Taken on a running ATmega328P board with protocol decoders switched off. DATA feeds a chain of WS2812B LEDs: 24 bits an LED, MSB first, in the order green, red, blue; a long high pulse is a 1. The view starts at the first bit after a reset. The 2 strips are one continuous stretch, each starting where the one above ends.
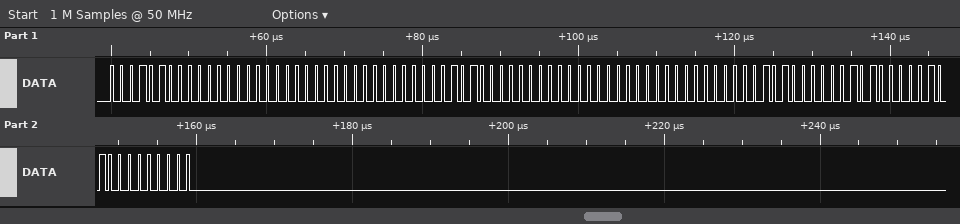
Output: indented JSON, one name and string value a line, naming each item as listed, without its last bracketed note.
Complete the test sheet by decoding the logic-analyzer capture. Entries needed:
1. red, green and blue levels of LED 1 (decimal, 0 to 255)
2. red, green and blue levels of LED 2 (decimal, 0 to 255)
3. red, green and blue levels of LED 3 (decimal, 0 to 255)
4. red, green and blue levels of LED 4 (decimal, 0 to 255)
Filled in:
{
  "red, green and blue levels of LED 1": "0, 20, 0",
  "red, green and blue levels of LED 2": "20, 0, 0",
  "red, green and blue levels of LED 3": "0, 0, 20",
  "red, green and blue levels of LED 4": "10, 10, 0"
}
